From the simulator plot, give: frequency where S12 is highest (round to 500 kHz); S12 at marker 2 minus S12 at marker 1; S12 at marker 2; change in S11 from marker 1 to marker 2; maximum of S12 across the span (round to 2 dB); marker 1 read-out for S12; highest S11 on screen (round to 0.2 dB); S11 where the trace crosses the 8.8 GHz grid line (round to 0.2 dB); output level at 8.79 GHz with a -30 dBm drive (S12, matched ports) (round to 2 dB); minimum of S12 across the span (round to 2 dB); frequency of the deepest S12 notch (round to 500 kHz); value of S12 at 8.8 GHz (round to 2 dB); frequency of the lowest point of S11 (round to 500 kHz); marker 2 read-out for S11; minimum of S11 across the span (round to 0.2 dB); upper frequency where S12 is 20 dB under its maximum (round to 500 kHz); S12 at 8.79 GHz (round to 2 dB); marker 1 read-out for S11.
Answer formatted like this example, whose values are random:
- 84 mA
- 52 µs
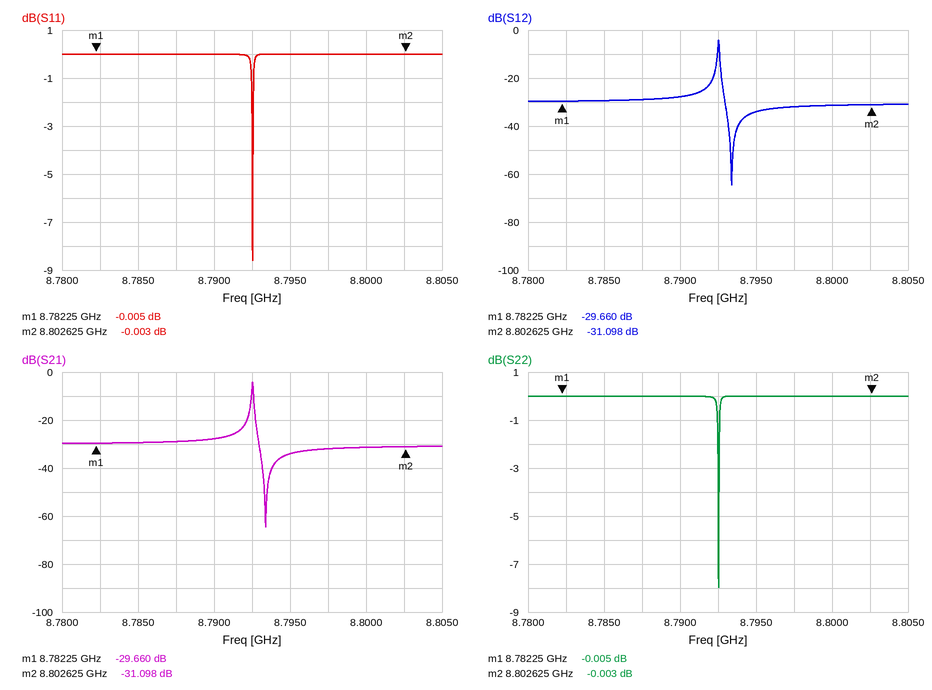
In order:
- 8.7925 GHz
- -1.438 dB
- -31.098 dB
- 0.002 dB
- -4 dB
- -29.660 dB
- 0.0 dB
- 0.0 dB
- -58 dBm
- -64 dB
- 8.7935 GHz
- -32 dB
- 8.7925 GHz
- -0.003 dB
- -8.6 dB
- 8.7930 GHz
- -28 dB
- -0.005 dB
